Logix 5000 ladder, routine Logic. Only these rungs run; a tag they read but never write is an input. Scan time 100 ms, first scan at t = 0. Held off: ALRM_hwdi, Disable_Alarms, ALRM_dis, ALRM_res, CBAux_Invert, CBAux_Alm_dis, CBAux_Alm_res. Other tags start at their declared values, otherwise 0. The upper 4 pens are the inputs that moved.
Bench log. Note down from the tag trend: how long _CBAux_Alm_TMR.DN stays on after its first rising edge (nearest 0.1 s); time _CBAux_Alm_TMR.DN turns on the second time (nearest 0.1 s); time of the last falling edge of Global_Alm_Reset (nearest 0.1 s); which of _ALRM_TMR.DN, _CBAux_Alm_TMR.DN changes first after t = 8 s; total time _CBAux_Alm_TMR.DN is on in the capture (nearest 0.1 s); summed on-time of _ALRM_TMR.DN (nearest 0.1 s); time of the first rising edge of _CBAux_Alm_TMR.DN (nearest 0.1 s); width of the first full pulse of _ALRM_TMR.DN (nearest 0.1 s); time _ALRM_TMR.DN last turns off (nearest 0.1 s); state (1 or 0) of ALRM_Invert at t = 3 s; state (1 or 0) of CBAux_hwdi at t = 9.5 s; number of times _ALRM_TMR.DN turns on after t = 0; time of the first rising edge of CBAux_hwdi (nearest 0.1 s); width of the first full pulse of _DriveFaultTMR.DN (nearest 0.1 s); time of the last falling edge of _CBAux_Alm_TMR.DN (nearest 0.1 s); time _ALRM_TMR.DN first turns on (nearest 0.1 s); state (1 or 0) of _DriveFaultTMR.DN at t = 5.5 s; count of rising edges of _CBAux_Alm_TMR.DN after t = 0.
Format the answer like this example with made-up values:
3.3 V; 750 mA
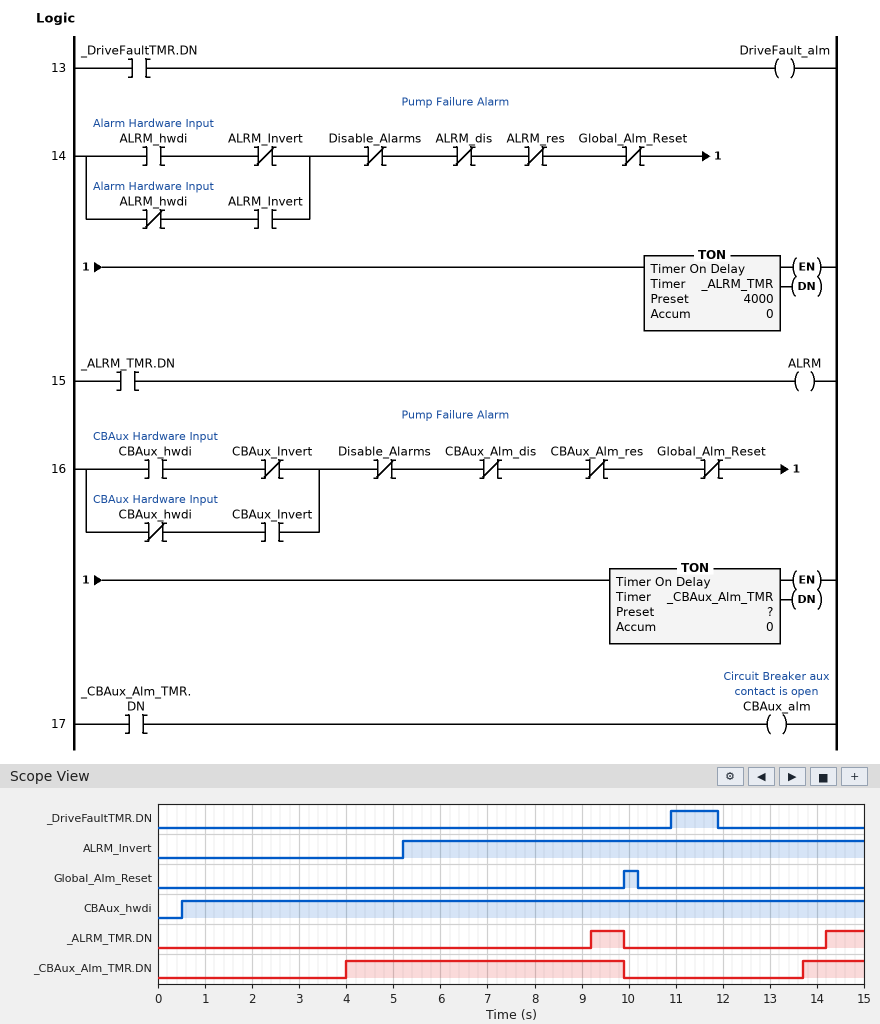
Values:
5.9 s; 13.7 s; 10.2 s; _ALRM_TMR.DN; 7.2 s; 1.5 s; 4.0 s; 0.7 s; 9.9 s; 0; 1; 2; 0.5 s; 1.0 s; 9.9 s; 9.2 s; 0; 2
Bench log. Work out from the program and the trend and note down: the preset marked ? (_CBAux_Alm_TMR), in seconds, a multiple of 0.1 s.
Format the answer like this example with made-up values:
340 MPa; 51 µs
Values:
3.5 s
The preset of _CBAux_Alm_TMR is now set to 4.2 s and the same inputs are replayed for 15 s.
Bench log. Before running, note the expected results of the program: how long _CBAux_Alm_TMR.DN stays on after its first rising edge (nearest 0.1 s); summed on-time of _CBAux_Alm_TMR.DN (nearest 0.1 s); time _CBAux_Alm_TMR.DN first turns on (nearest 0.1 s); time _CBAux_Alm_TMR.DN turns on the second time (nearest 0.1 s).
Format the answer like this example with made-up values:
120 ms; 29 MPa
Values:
5.2 s; 5.8 s; 4.7 s; 14.4 s
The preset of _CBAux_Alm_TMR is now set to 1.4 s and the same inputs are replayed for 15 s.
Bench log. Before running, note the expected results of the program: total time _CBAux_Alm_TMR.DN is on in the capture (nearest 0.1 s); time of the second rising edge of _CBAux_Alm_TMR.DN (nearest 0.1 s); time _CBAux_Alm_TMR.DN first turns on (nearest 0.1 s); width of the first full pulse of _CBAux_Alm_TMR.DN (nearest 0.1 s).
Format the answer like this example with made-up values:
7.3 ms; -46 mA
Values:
11.4 s; 11.6 s; 1.9 s; 8.0 s
